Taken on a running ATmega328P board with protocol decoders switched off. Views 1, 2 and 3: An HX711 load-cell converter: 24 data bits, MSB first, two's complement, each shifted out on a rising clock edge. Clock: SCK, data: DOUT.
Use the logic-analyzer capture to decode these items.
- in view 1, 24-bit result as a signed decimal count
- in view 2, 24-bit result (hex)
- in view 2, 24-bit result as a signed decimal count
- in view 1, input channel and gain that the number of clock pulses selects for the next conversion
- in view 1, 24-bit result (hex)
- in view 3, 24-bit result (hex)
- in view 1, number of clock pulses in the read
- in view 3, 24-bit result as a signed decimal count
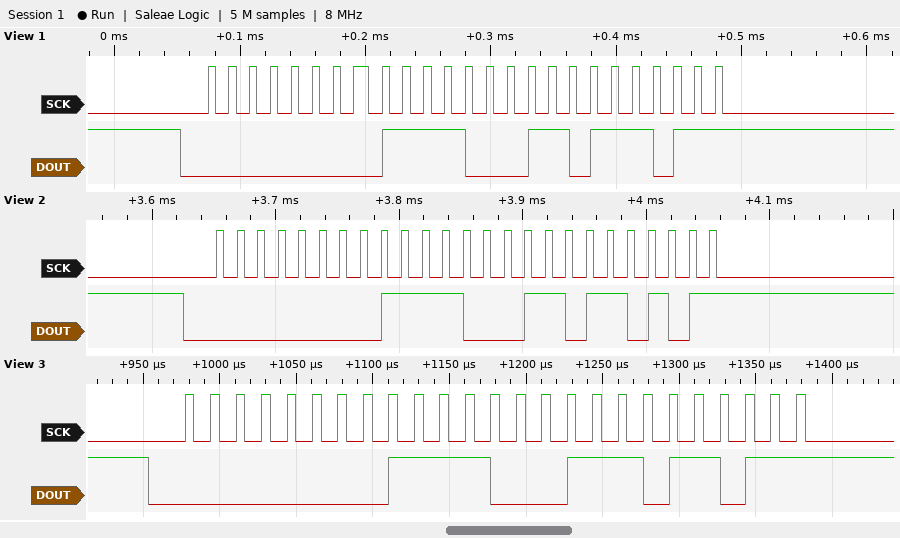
61883
0x00F1B5
61877
channel A, gain 128
0x00F1BB
0x00F1DB
25
61915
